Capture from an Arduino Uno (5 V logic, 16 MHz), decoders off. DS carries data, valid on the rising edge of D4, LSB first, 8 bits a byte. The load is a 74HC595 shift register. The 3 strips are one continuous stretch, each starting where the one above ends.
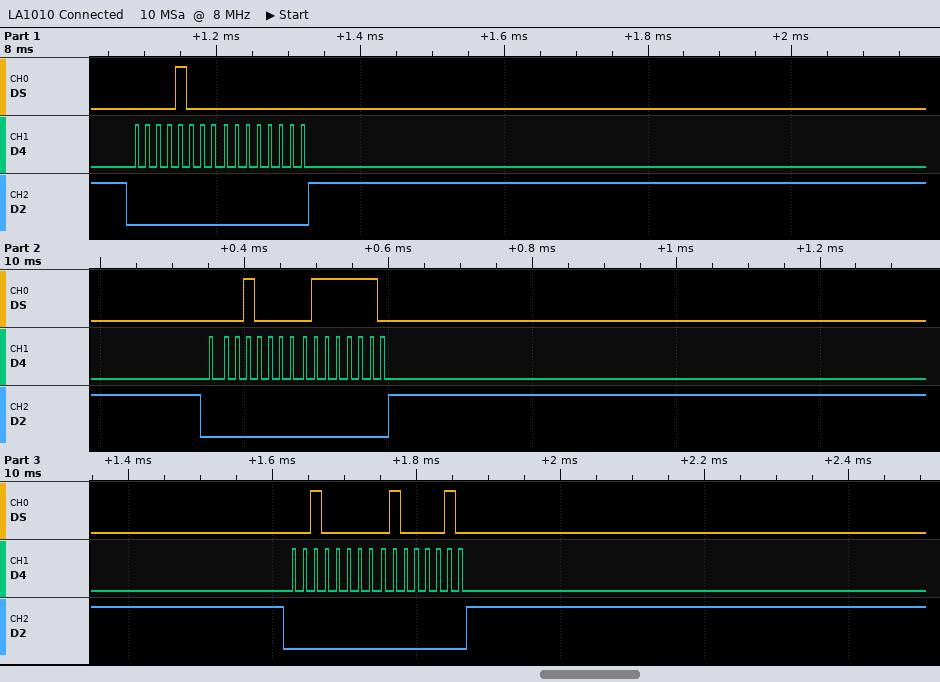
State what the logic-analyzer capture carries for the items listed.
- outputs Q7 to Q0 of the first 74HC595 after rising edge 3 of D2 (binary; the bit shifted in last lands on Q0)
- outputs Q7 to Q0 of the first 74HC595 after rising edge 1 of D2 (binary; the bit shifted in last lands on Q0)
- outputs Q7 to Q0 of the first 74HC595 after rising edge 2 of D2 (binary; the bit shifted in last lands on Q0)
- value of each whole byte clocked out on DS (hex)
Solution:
01000010
00000000
01111110
0x10 0x00 0x08 0x7E 0x04 0x42
